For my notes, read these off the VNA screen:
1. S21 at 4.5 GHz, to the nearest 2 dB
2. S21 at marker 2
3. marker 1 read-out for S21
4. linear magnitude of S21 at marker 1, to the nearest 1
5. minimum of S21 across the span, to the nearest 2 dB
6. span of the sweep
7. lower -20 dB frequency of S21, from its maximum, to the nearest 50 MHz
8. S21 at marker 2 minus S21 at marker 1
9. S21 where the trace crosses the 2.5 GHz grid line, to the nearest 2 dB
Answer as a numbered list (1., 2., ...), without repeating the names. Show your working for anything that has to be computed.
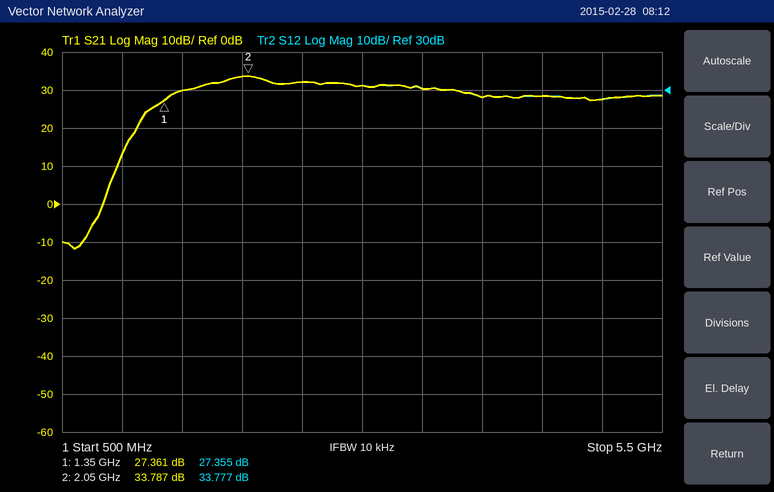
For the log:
1. 28 dB
2. 33.787 dB
3. 27.361 dB
4. 10^(27.361/20) ≈ 23
5. -12 dB
6. 5 GHz
7. 1.00 GHz
8. 33.787 − (27.361) = 6.426 dB
9. 32 dB
